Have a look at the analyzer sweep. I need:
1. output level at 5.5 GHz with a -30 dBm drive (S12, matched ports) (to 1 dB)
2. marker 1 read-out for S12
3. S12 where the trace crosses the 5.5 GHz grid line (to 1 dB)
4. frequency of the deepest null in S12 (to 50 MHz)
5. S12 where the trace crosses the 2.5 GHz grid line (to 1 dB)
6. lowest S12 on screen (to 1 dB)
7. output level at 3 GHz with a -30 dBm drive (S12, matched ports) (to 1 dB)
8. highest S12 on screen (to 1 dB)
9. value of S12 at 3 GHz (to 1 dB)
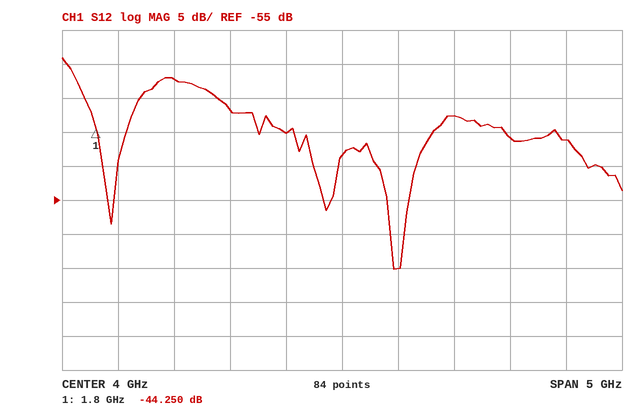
-76 dBm
-44.250 dB
-46 dB
4.45 GHz
-37 dB
-65 dB
-72 dBm
-34 dB
-42 dB
